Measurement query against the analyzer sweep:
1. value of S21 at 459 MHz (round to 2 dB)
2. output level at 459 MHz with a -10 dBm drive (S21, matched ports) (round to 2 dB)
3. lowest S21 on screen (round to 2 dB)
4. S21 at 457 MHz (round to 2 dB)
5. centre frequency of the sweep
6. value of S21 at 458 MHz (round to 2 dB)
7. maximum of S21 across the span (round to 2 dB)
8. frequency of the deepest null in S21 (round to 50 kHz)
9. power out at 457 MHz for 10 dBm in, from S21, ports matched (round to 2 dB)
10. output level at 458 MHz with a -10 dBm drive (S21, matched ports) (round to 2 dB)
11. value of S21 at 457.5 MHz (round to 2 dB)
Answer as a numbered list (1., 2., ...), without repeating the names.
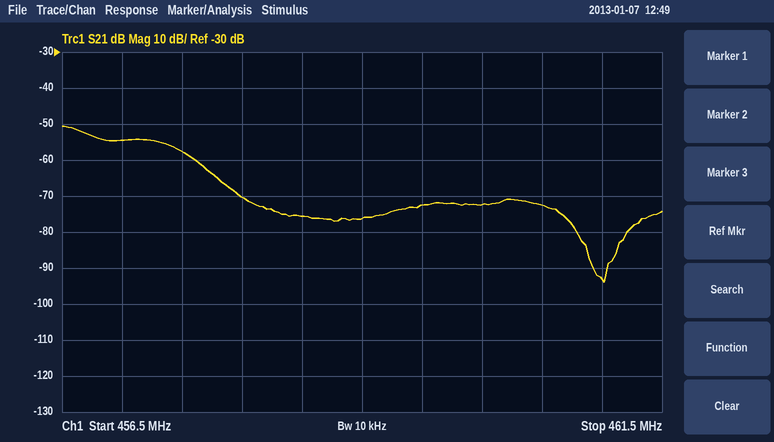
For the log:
1. -76 dB
2. -86 dBm
3. -94 dB
4. -54 dB
5. 459 MHz
6. -70 dB
7. -50 dB
8. 461.00 MHz
9. -44 dBm
10. -80 dBm
11. -58 dB
